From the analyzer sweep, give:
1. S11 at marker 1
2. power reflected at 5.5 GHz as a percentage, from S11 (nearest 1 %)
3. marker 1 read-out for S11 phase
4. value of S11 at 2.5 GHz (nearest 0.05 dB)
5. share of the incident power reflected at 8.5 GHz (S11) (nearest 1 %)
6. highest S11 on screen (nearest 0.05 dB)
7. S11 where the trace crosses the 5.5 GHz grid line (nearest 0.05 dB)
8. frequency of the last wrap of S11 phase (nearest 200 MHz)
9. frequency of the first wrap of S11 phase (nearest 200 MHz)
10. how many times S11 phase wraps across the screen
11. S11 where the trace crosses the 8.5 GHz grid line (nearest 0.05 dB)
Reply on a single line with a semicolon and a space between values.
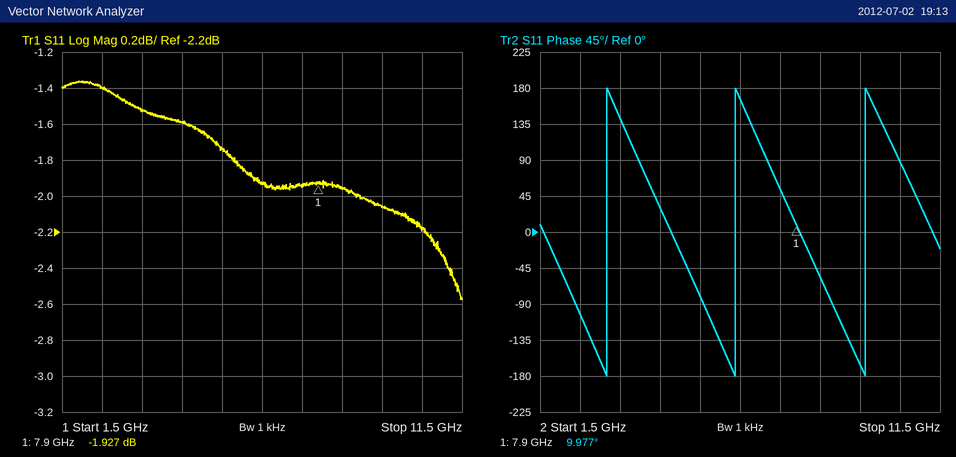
-1.927 dB; 67 %; 9.977°; -1.40 dB; 64 %; -1.35 dB; -1.75 dB; 9.6 GHz; 3.2 GHz; 3; -1.95 dB
